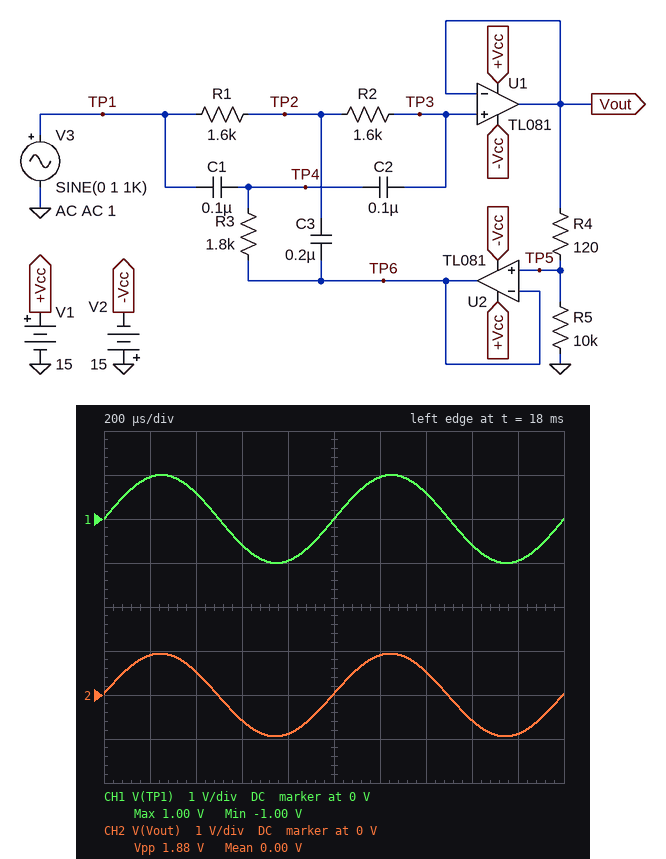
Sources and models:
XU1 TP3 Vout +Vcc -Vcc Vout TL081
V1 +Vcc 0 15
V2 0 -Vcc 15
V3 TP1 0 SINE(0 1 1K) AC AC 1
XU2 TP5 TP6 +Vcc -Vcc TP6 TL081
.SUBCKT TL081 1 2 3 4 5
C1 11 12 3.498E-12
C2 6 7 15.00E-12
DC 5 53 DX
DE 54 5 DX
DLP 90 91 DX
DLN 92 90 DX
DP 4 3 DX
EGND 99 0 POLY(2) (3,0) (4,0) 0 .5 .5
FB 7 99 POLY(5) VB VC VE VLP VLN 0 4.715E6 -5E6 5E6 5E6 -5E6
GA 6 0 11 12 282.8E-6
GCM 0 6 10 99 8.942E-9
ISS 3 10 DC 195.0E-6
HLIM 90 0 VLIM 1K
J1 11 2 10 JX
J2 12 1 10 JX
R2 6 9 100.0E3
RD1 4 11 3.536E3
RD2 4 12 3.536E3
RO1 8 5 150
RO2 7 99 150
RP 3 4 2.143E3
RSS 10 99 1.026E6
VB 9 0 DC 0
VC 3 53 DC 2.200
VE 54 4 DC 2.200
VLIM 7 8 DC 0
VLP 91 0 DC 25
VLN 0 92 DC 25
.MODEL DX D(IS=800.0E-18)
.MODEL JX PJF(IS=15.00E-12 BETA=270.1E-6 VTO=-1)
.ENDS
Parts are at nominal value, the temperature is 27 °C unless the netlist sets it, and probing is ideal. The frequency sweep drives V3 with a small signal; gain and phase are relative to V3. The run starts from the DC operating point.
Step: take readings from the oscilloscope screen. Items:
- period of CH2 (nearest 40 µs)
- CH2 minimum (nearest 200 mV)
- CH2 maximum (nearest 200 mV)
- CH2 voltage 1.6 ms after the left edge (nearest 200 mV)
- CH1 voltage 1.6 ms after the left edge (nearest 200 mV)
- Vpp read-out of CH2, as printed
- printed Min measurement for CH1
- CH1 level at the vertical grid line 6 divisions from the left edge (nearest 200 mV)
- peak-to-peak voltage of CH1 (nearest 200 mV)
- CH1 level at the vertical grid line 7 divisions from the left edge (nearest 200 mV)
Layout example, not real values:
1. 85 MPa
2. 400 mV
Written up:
1. 1.00 ms
2. -1.0 V
3. 1.0 V
4. -600 mV
5. -600 mV
6. 1.88 V
7. -1.00 V
8. 1.0 V
9. 2.0 V
10. 600 mV
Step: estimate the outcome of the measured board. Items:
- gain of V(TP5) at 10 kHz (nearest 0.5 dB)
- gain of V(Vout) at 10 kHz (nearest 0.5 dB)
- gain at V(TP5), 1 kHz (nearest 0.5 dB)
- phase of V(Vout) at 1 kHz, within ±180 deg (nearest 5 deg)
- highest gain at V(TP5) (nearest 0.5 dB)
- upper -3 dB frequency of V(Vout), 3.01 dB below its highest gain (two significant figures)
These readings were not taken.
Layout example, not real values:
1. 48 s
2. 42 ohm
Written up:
1. 0 dB
2. 0 dB
3. -0.5 dB
4. 0 deg
5. 0 dB
6. 4.8 MHz
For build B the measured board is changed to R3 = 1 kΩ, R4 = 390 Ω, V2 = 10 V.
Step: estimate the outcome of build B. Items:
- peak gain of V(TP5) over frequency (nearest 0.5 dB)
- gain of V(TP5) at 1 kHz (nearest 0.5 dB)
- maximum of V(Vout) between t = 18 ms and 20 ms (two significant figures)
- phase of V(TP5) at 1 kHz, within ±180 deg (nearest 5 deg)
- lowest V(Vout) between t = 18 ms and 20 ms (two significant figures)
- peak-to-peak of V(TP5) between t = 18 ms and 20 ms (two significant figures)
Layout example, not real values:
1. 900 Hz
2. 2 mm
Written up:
1. -0.5 dB
2. -5.0 dB
3. 580 mV
4. 20 deg
5. -580 mV
6. 1.1 V
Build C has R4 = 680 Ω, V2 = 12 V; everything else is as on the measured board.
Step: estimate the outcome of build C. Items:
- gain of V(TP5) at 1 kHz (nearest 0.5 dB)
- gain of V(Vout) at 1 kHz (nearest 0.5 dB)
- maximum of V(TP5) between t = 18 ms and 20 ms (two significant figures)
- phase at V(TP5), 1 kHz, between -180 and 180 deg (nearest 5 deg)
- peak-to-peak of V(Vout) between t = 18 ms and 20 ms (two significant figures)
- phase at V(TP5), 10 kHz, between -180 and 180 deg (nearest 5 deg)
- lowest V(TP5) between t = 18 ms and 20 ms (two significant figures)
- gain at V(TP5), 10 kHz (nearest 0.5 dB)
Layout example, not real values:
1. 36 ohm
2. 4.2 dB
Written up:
1. -3.0 dB
2. -2.5 dB
3. 700 mV
4. 10 deg
5. 1.5 V
6. 0 deg
7. -700 mV
8. -0.5 dB
